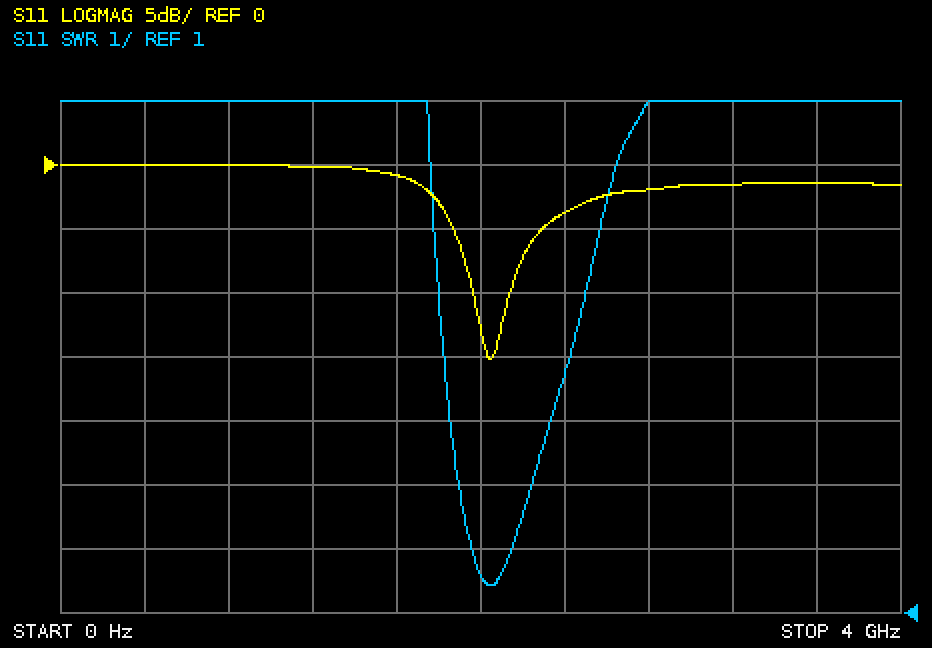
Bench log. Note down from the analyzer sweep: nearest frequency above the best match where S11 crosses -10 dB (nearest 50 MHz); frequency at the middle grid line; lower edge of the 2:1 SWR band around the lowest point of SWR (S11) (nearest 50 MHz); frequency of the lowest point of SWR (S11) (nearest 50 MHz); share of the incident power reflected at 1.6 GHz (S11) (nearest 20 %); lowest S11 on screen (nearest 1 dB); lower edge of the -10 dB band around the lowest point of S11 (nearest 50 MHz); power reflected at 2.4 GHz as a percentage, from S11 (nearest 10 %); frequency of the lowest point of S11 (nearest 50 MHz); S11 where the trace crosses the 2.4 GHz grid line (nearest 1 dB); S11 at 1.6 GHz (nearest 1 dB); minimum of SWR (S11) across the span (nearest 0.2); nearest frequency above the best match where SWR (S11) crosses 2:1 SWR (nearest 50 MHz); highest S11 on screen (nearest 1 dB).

2.15 GHz
2 GHz
1.95 GHz
2.05 GHz
80 %
-15 dB
1.95 GHz
40 %
2.05 GHz
-4 dB
-1 dB
1.4
2.15 GHz
0 dB
